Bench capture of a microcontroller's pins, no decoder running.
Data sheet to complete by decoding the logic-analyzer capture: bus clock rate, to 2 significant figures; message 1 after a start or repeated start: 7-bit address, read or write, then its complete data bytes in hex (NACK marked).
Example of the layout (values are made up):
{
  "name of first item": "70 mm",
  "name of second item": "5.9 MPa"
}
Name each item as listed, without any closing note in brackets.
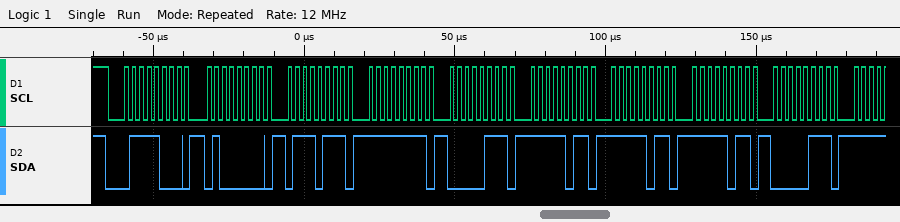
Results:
{
  "bus clock rate, to 2 significant figures": "400 kHz",
  "message 1 after a start or repeated start: 7-bit address, read or write, then its complete data bytes in hex": "0x3C write: 40 77 FF 07 FB FB FB 07"
}
